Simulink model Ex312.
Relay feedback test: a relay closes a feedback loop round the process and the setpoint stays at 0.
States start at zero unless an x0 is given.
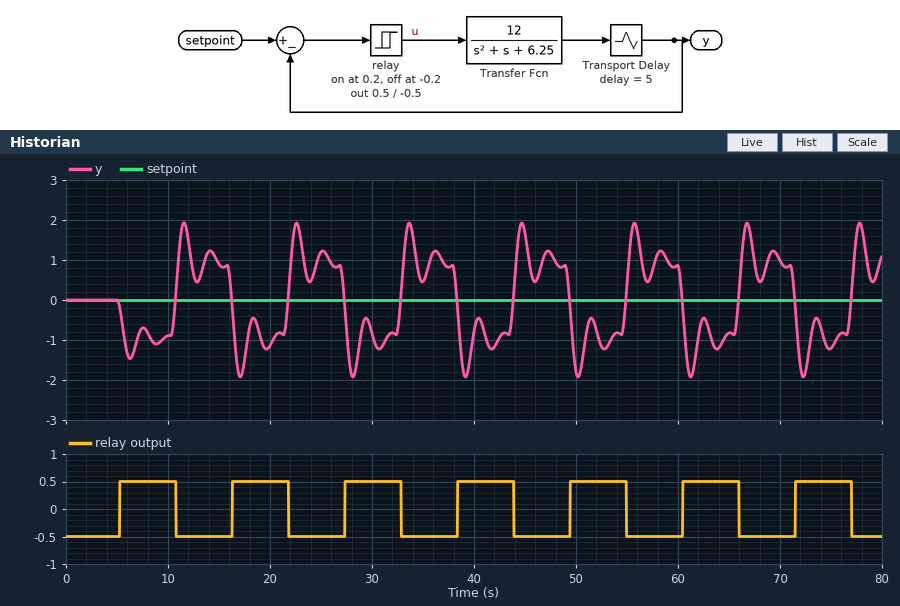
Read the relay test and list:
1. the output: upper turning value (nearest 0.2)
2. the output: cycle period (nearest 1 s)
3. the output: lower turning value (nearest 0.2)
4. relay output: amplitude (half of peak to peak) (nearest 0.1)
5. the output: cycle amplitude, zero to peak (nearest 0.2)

2.0
11 s
-2.0
0.5
2.0
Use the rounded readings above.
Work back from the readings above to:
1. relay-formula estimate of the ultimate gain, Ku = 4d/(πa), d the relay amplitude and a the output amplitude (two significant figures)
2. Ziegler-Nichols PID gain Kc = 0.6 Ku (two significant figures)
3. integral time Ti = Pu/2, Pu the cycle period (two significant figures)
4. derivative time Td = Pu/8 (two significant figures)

0.32
0.19
5.5 s
1.4 s
